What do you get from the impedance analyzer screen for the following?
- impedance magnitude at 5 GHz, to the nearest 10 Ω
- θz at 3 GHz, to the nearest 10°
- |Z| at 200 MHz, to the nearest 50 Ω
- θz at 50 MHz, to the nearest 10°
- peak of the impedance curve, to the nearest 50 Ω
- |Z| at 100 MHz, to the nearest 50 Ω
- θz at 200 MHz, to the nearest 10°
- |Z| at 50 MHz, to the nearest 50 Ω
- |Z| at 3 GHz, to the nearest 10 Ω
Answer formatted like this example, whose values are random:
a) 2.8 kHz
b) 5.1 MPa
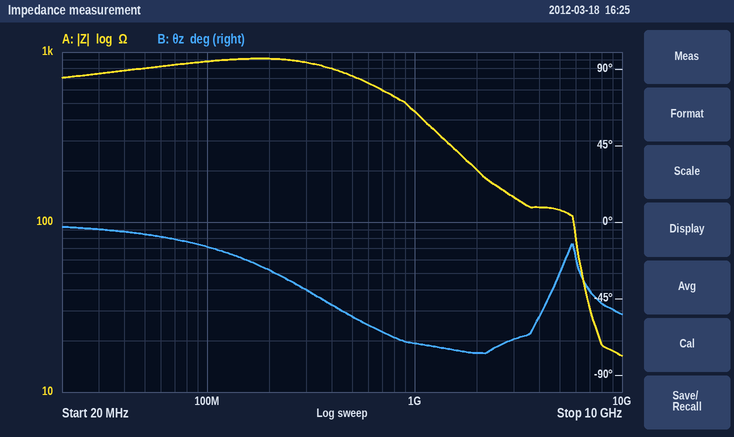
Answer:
a) 120 Ω
b) -70°
c) 900 Ω
d) -10°
e) 900 Ω
f) 900 Ω
g) -30°
h) 800 Ω
i) 140 Ω
